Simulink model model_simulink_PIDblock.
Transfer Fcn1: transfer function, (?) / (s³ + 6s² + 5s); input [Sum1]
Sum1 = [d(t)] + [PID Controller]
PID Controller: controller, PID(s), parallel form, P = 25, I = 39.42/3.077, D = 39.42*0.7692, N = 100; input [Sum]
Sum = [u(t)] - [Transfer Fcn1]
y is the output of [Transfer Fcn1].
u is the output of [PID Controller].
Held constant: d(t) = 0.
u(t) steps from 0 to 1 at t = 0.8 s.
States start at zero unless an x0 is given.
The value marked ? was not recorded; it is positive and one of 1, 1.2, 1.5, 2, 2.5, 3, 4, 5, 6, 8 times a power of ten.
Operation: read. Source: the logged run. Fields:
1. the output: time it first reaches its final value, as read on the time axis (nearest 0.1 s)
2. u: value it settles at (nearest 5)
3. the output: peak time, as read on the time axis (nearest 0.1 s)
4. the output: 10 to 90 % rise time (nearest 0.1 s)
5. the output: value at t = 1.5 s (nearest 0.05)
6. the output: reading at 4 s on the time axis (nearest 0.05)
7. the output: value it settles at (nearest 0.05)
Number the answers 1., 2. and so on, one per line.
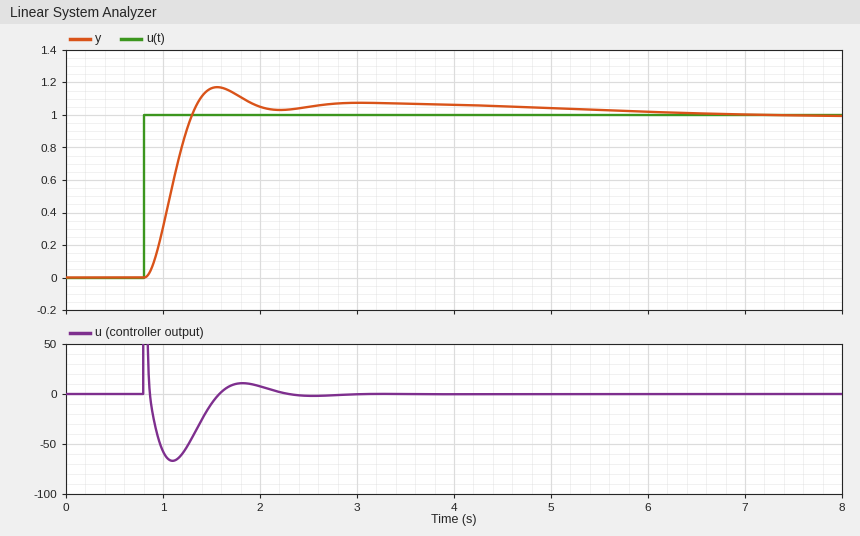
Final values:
1. 1.3 s
2. 0
3. 1.6 s
4. 0.3 s
5. 1.15
6. 1.05
7. 1.00
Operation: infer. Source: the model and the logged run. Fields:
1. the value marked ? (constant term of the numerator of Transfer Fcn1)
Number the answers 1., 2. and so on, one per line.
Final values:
1. 0.8
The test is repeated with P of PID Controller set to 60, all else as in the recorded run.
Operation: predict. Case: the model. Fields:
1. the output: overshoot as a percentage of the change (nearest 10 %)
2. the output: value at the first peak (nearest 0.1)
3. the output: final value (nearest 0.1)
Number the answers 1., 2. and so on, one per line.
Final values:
1. 40 %
2. 1.4
3. 1.0
